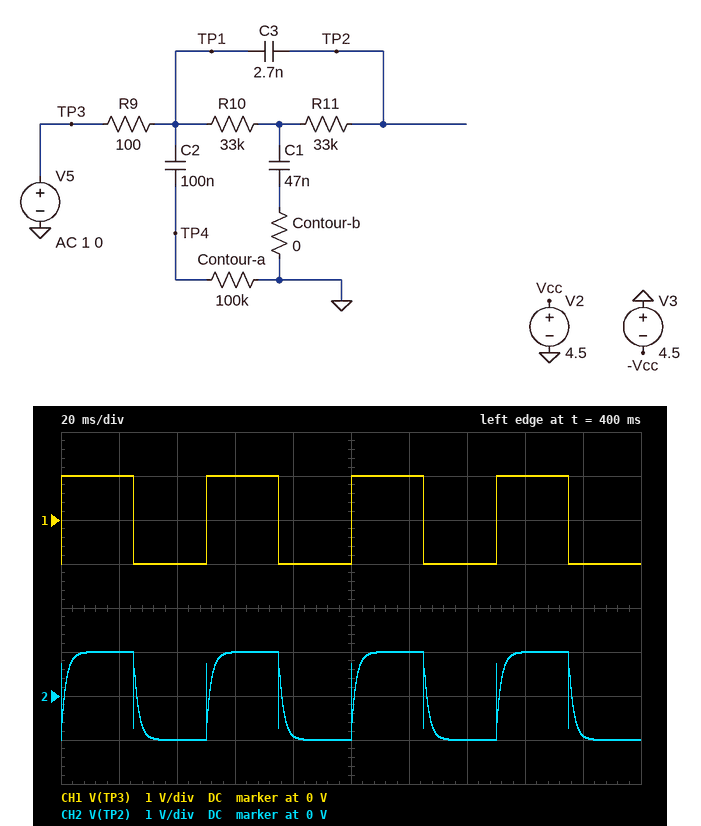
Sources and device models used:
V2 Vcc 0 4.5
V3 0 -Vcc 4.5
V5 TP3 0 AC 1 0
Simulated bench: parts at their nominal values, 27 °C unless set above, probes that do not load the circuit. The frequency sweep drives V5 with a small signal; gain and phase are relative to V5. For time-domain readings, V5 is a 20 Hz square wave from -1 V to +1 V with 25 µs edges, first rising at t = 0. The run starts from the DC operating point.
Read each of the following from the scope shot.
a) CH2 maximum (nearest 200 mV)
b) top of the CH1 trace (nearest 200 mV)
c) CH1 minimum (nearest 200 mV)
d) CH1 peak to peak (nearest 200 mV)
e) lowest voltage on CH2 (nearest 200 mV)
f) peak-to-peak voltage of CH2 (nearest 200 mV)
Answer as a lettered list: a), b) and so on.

a) 1.0 V
b) 1.0 V
c) -1.0 V
d) 2.0 V
e) -1.0 V
f) 2.0 V
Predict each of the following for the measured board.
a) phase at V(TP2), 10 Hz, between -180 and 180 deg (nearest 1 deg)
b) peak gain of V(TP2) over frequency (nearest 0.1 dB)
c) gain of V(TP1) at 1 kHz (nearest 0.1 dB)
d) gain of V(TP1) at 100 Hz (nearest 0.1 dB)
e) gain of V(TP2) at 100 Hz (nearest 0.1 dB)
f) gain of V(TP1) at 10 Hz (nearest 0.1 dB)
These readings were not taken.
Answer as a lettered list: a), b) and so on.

a) -6 deg
b) 0 dB
c) 0 dB
d) 0 dB
e) -3.6 dB
f) 0 dB
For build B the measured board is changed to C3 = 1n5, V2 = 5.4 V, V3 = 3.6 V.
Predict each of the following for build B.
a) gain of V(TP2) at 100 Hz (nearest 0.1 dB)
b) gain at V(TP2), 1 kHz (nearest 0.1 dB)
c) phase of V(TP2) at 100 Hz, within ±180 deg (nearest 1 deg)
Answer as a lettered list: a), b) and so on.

a) -3.3 dB
b) -14.0 dB
c) -43 deg
